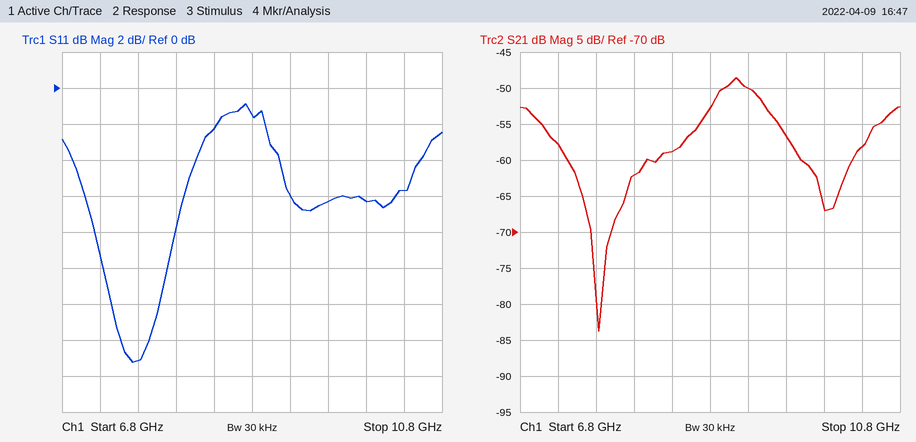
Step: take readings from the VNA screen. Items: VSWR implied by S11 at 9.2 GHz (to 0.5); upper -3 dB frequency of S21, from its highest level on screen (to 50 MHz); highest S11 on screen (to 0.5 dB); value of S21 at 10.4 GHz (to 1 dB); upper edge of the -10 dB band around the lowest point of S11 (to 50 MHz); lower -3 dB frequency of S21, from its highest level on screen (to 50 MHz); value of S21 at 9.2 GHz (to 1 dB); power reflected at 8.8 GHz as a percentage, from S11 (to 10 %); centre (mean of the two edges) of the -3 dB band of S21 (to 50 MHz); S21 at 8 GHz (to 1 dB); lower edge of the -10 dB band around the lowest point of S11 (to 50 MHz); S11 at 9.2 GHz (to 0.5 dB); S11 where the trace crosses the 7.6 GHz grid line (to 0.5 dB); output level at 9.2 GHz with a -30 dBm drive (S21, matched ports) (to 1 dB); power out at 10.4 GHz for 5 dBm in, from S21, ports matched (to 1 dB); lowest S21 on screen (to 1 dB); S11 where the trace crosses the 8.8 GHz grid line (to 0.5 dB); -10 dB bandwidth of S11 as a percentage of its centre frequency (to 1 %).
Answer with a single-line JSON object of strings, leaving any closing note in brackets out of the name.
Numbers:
{"VSWR implied by S11 at 9.2 GHz": "3.0", "upper -3 dB frequency of S21, from its highest level on screen": "9.35 GHz", "highest S11 on screen": "-1.0 dB", "value of S21 at 10.4 GHz": "-58 dB", "upper edge of the -10 dB band around the lowest point of S11": "7.90 GHz", "lower -3 dB frequency of S21, from its highest level on screen": "8.85 GHz", "value of S21 at 9.2 GHz": "-50 dB", "power reflected at 8.8 GHz as a percentage, from S11": "70 %", "centre (mean of the two edges) of the -3 dB band of S21": "9.10 GHz", "S21 at 8 GHz": "-62 dB", "lower edge of the -10 dB band around the lowest point of S11": "7.25 GHz", "S11 at 9.2 GHz": "-6.0 dB", "S11 where the trace crosses the 7.6 GHz grid line": "-15.0 dB", "output level at 9.2 GHz with a -30 dBm drive (S21, matched ports)": "-80 dBm", "power out at 10.4 GHz for 5 dBm in, from S21, ports matched": "-53 dBm", "lowest S21 on screen": "-84 dB", "S11 where the trace crosses the 8.8 GHz grid line": "-1.5 dB", "-10 dB bandwidth of S11 as a percentage of its centre frequency": "9 %"}
